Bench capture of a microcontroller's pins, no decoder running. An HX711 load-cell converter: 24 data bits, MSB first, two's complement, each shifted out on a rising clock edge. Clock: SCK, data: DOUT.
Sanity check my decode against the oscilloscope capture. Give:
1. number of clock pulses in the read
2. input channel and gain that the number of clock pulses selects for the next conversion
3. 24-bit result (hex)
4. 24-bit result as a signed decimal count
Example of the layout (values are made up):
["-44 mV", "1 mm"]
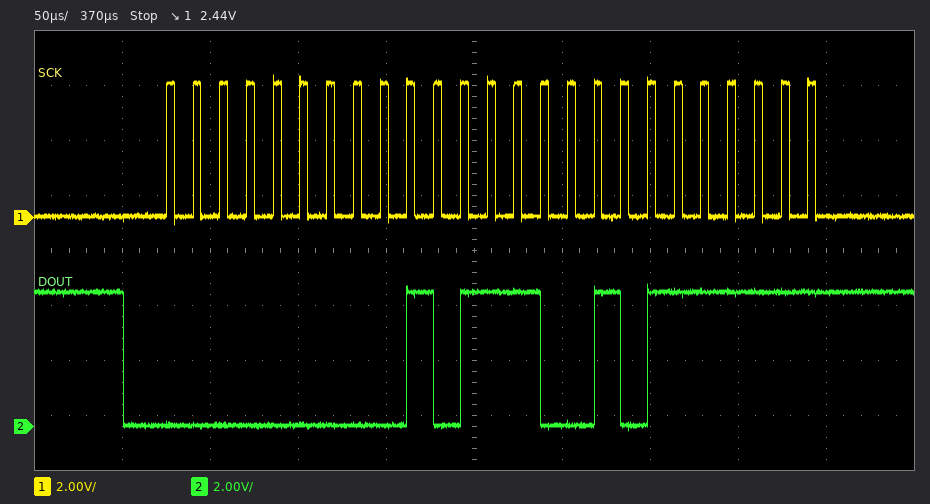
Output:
["25", "channel A, gain 128", "0x005CBF", "23743"]
